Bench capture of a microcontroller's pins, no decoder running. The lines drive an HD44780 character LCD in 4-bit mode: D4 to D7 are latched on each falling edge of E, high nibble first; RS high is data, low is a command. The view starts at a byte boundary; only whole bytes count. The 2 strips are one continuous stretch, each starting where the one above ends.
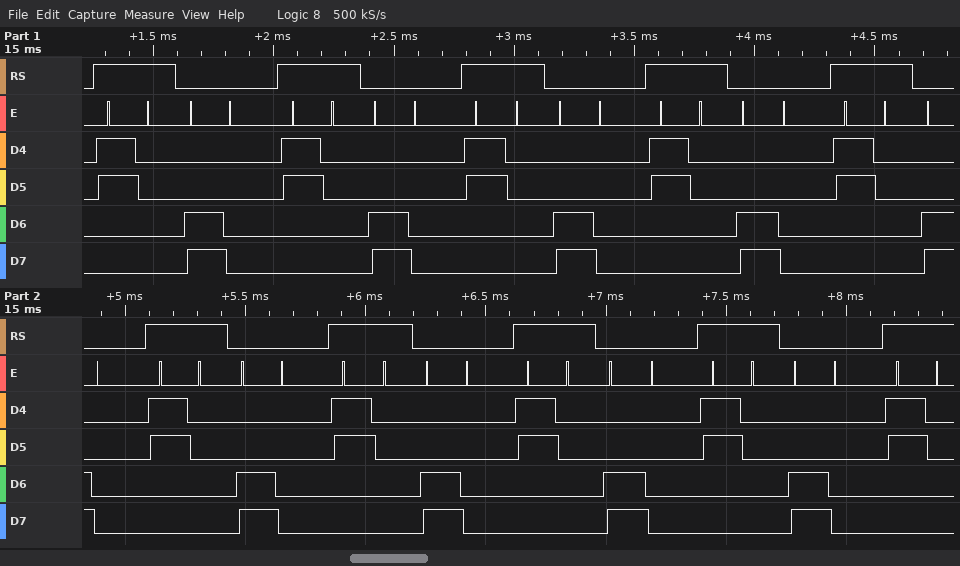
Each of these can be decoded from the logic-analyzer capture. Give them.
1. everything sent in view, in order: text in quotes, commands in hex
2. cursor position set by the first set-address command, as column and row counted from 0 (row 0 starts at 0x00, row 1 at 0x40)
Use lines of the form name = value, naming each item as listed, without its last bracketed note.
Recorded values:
everything sent in view, in order: text in quotes, commands in hex = "0" 0xC0 "0" 0xC0 "0" 0xC0 "0" 0xC0 "0" 0xC0 "0" 0xC0 "0" 0xC0 "0" 0xC0 "0" 0xC0 "0"
cursor position set by the first set-address command, as column and row counted from 0 = column 0, row 1
